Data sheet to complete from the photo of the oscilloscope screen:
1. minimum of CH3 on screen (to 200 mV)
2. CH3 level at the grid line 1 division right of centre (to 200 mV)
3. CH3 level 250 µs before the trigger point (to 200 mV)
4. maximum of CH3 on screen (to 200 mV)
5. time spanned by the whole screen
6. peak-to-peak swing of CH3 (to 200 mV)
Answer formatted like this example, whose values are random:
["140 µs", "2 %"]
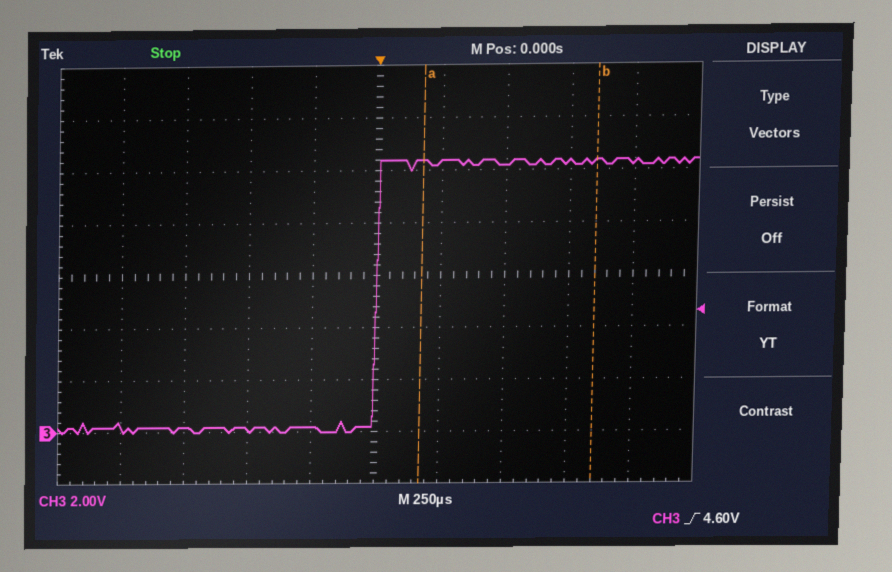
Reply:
["0.0 V", "10.4 V", "200 mV", "10.4 V", "2.5 ms", "10.4 V"]
